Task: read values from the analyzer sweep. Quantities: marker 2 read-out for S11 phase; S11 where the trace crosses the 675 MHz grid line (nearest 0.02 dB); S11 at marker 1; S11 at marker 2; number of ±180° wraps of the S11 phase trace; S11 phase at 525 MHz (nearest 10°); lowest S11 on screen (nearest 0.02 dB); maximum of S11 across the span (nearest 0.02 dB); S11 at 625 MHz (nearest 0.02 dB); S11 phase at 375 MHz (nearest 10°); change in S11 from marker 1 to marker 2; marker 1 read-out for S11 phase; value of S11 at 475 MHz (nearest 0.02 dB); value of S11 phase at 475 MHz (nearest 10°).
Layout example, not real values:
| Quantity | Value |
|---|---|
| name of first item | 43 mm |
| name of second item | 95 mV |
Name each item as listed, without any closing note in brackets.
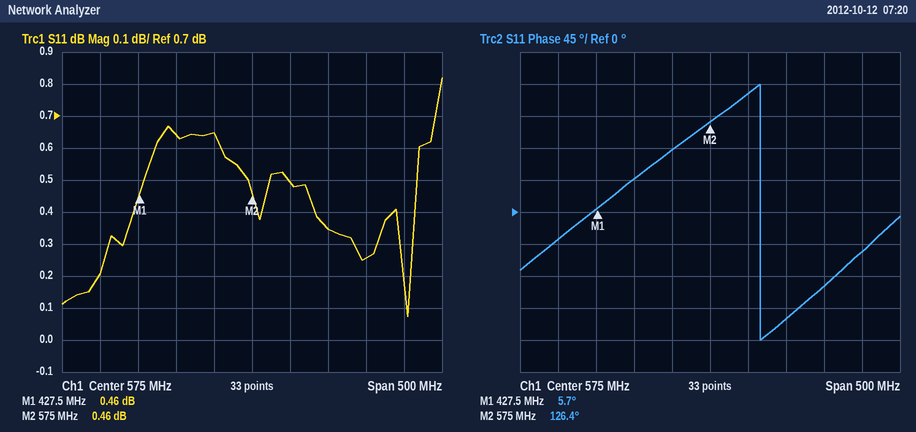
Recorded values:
| Quantity | Value |
|---|---|
| marker 2 read-out for S11 phase | 126.4° |
| S11 where the trace crosses the 675 MHz grid line | 0.34 dB |
| S11 at marker 1 | 0.46 dB |
| S11 at marker 2 | 0.46 dB |
| number of ±180° wraps of the S11 phase trace | 1 |
| S11 phase at 525 MHz | 90° |
| lowest S11 on screen | 0.08 dB |
| maximum of S11 across the span | 0.82 dB |
| S11 at 625 MHz | 0.50 dB |
| S11 phase at 375 MHz | -40° |
| change in S11 from marker 1 to marker 2 | 0.00 dB |
| marker 1 read-out for S11 phase | 5.7° |
| value of S11 at 475 MHz | 0.64 dB |
| value of S11 phase at 475 MHz | 50° |
